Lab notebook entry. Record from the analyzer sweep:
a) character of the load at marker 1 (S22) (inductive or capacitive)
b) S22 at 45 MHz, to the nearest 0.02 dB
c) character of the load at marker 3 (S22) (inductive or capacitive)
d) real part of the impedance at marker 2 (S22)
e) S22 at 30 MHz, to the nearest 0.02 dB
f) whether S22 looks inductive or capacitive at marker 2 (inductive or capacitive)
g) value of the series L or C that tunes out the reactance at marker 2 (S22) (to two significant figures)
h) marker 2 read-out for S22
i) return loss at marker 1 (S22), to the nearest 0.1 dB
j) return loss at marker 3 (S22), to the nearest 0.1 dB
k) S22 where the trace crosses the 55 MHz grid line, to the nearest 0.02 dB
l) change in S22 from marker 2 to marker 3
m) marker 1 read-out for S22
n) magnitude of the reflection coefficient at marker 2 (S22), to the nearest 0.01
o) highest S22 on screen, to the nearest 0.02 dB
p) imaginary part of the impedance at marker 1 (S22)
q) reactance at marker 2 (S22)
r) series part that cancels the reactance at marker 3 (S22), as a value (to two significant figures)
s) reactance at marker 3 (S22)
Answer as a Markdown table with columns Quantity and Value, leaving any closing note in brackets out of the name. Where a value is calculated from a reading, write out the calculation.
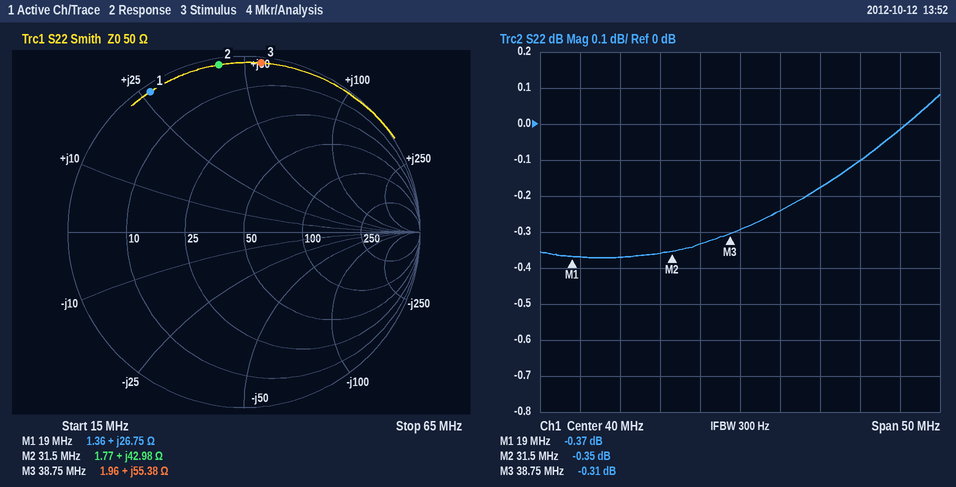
| Quantity | Value |
|---|---|
| character of the load at marker 1 (S22) | inductive |
| S22 at 45 MHz, to the nearest 0.02 dB | -0.24 dB |
| character of the load at marker 3 (S22) | inductive |
| real part of the impedance at marker 2 | 1.77 Ω |
| S22 at 30 MHz, to the nearest 0.02 dB | -0.36 dB |
| whether S22 looks inductive or capacitive at marker 2 | inductive |
| value of the series L or C that tunes out the reactance at marker 2 (S22) | C = 1/(2π × 31.5 MHz × 42.98 Ω) ≈ 118 pF, so 120 pF to two significant figures |
| marker 2 read-out for S22 | -0.35 dB |
| return loss at marker 1 (S22), to the nearest 0.1 dB | 0.4 dB |
| return loss at marker 3 (S22), to the nearest 0.1 dB | 0.3 dB |
| S22 where the trace crosses the 55 MHz grid line, to the nearest 0.02 dB | -0.10 dB |
| change in S22 from marker 2 to marker 3 | -0.31 − (-0.35) = 0.04 dB |
| marker 1 read-out for S22 | -0.37 dB |
| magnitude of the reflection coefficient at marker 2 (S22), to the nearest 0.01 | 0.96 |
| highest S22 on screen, to the nearest 0.02 dB | 0.08 dB |
| imaginary part of the impedance at marker 1 | +26.75 Ω |
| reactance at marker 2 | +42.98 Ω |
| series part that cancels the reactance at marker 3 (S22), as a value | C = 1/(2π × 38.75 MHz × 55.38 Ω) ≈ 74 pF |
| reactance at marker 3 | +55.38 Ω |
